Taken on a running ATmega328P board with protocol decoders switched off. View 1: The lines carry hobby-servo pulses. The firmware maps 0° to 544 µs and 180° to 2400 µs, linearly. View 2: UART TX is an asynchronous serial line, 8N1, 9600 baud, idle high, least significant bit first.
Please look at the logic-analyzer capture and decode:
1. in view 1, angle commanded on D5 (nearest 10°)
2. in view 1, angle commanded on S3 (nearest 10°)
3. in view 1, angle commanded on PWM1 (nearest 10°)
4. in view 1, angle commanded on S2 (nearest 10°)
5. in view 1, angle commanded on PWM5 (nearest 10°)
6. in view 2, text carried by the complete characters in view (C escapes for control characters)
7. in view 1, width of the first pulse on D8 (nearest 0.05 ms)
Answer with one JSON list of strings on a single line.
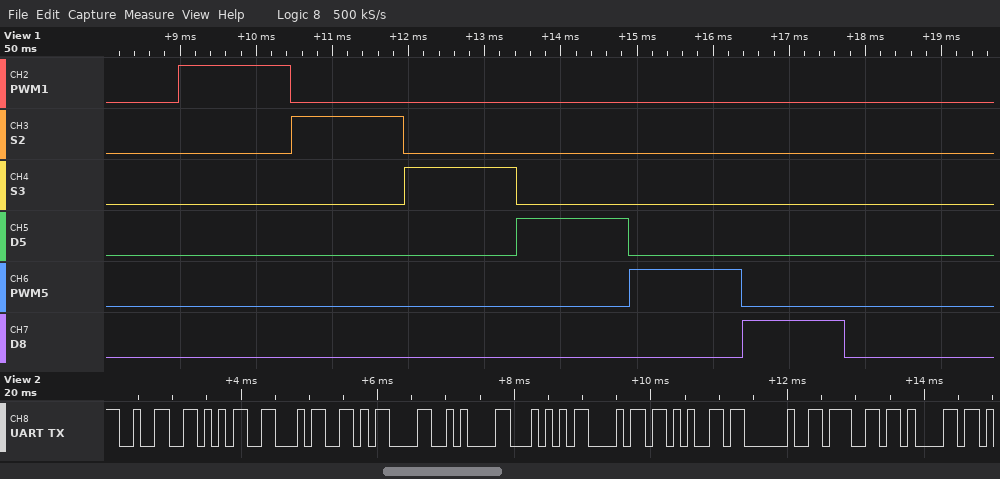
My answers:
["90°", "90°", "90°", "90°", "90°", "\"254\\r\\nThe ga\"", "1.35 ms"]
